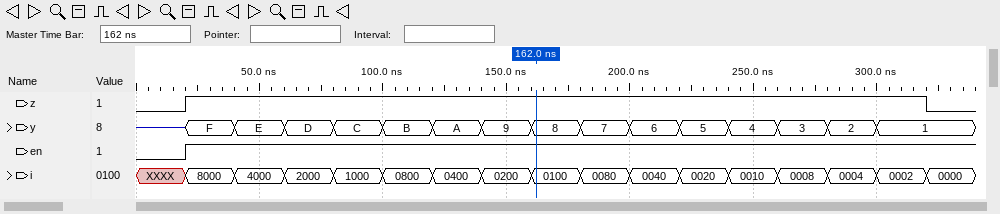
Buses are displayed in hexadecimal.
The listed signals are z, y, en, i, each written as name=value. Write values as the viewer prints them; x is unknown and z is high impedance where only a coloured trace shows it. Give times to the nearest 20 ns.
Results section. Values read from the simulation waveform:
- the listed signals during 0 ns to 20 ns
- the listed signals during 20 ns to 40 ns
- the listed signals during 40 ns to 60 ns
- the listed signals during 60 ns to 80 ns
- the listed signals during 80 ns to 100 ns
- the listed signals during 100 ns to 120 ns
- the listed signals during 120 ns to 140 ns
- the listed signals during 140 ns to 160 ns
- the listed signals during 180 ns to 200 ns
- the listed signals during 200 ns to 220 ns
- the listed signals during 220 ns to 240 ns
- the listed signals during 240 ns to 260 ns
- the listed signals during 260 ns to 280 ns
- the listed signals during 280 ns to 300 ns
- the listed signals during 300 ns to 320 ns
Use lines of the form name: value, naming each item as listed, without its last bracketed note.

the listed signals during 0 ns to 20 ns: z=0, y=z, en=0, i=XXXX
the listed signals during 20 ns to 40 ns: z=1, y=F, en=1, i=8000
the listed signals during 40 ns to 60 ns: z=1, y=E, en=1, i=4000
the listed signals during 60 ns to 80 ns: z=1, y=D, en=1, i=2000
the listed signals during 80 ns to 100 ns: z=1, y=C, en=1, i=1000
the listed signals during 100 ns to 120 ns: z=1, y=B, en=1, i=0800
the listed signals during 120 ns to 140 ns: z=1, y=A, en=1, i=0400
the listed signals during 140 ns to 160 ns: z=1, y=9, en=1, i=0200
the listed signals during 180 ns to 200 ns: z=1, y=7, en=1, i=0080
the listed signals during 200 ns to 220 ns: z=1, y=6, en=1, i=0040
the listed signals during 220 ns to 240 ns: z=1, y=5, en=1, i=0020
the listed signals during 240 ns to 260 ns: z=1, y=4, en=1, i=0010
the listed signals during 260 ns to 280 ns: z=1, y=3, en=1, i=0008
the listed signals during 280 ns to 300 ns: z=1, y=2, en=1, i=0004
the listed signals during 300 ns to 320 ns: z=1, y=1, en=1, i=0002
